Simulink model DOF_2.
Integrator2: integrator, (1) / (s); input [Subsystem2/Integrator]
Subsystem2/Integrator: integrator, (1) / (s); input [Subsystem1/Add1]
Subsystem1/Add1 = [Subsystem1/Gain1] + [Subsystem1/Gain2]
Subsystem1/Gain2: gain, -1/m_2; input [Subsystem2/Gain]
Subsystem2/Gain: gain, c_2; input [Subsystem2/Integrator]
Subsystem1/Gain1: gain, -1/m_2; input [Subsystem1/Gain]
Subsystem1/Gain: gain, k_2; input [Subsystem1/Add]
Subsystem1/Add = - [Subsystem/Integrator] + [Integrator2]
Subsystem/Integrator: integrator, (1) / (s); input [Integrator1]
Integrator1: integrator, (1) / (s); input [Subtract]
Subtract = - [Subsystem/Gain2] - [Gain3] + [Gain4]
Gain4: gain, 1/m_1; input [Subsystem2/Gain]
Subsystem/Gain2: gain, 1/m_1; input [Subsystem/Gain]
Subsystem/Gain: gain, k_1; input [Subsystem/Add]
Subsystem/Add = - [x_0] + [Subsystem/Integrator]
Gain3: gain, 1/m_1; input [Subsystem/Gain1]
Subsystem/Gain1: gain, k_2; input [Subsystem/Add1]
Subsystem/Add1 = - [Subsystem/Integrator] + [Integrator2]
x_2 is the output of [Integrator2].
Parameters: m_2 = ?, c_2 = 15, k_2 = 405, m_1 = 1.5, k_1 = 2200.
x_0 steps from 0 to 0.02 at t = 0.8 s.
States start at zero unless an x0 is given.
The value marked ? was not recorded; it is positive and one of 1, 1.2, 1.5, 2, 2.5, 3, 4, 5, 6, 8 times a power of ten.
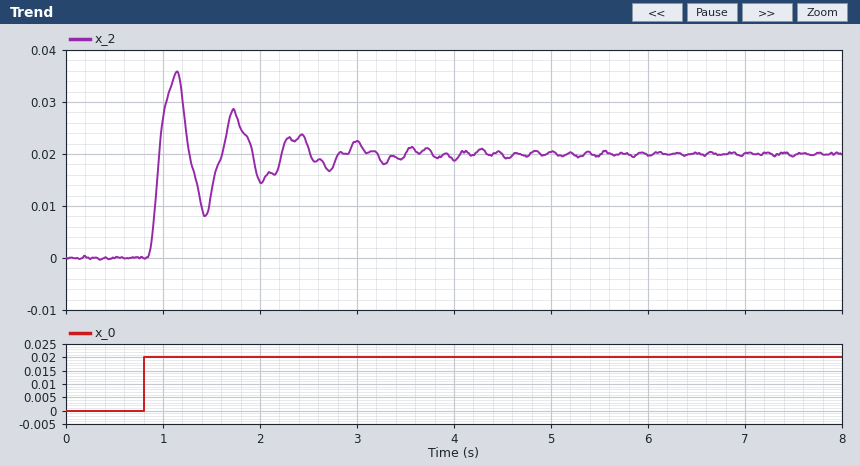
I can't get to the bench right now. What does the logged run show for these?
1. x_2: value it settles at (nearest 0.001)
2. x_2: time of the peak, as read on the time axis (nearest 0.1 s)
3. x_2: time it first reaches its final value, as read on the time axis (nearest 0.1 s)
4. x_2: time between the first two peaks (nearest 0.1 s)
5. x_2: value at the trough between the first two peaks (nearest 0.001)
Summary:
0.020
1.1 s
1.0 s
0.6 s
0.008
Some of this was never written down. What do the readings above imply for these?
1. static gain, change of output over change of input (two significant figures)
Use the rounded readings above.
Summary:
1.0
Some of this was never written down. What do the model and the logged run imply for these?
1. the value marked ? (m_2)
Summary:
5
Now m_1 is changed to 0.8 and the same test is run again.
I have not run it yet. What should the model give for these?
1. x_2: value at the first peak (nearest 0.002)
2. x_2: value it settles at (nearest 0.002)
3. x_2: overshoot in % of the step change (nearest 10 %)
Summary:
0.034
0.020
70 %
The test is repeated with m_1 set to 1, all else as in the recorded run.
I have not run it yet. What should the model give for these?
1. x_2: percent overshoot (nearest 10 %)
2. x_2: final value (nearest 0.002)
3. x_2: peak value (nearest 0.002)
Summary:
80 %
0.020
0.036
